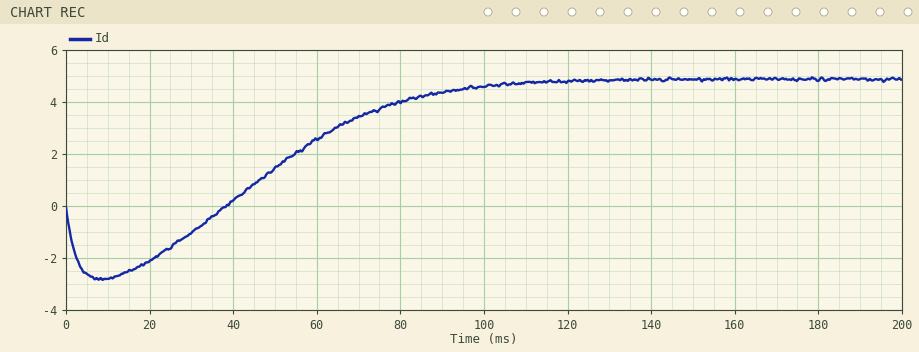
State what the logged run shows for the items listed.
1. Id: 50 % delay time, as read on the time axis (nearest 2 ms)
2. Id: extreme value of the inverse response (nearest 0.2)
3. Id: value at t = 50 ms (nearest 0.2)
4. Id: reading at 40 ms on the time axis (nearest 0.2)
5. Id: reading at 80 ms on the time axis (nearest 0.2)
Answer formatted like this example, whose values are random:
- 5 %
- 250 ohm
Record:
- 58 ms
- -2.8
- 1.4
- 0.2
- 4.0
